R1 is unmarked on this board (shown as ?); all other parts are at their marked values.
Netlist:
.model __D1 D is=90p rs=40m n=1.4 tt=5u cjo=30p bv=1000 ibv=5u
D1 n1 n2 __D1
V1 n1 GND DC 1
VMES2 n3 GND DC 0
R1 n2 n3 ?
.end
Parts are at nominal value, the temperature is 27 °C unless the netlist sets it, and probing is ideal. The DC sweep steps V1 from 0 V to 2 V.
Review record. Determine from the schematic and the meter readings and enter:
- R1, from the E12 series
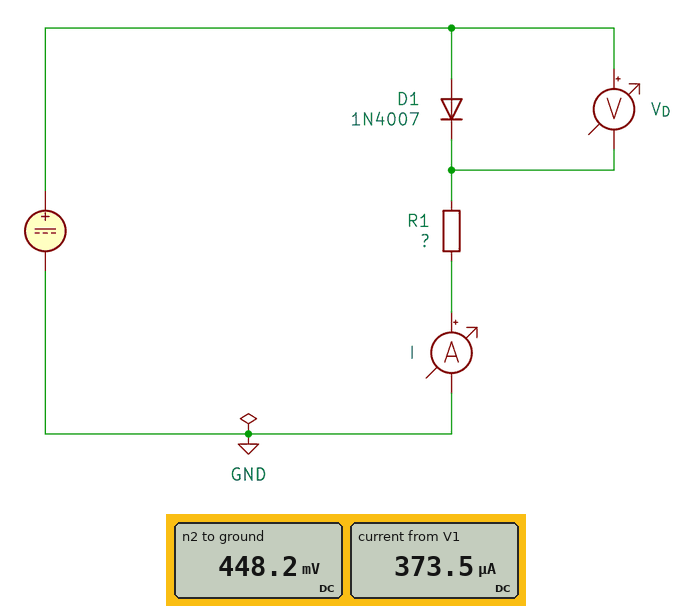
1.2 kΩ
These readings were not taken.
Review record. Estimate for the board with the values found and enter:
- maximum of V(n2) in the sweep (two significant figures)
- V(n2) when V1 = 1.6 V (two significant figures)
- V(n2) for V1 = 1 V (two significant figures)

1.4 V
1.0 V
450 mV
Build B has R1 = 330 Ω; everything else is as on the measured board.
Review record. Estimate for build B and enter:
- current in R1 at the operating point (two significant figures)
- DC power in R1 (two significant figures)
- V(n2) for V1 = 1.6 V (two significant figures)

1.2 mA
500 µW
970 mV
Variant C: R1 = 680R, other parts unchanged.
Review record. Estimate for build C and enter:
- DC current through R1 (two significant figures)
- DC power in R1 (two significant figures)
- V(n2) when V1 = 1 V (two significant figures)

630 µA
270 µW
430 mV
